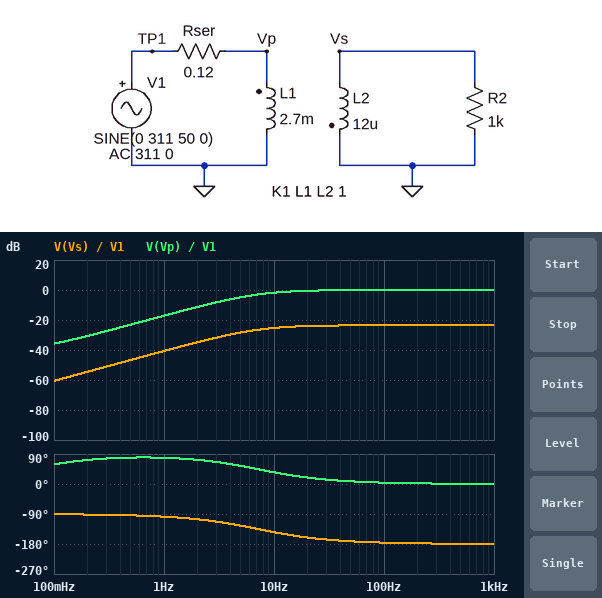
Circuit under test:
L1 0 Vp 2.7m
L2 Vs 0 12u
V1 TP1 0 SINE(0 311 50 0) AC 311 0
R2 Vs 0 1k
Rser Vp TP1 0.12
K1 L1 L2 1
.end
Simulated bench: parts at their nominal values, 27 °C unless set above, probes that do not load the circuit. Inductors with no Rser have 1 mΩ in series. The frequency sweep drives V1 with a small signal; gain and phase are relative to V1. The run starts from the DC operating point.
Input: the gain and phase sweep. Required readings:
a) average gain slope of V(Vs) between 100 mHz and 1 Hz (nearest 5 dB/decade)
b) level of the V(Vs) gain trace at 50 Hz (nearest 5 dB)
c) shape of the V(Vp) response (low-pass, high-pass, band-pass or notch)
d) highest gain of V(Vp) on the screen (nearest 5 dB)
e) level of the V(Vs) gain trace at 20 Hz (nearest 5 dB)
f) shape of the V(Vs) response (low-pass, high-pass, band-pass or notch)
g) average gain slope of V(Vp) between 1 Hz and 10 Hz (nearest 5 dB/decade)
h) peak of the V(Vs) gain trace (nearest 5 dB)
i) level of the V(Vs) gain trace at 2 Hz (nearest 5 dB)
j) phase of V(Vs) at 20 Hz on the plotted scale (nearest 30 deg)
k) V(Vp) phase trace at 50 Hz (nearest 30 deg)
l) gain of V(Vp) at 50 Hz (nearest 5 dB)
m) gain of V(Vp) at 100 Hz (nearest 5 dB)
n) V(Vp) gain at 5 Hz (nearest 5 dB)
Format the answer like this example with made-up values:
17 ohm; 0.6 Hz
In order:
20 dB/decade; -25 dB; high-pass; 0 dB; -25 dB; high-pass; 15 dB/decade; -25 dB; -35 dB; -150 deg; 0 deg; 0 dB; 0 dB; -5 dB
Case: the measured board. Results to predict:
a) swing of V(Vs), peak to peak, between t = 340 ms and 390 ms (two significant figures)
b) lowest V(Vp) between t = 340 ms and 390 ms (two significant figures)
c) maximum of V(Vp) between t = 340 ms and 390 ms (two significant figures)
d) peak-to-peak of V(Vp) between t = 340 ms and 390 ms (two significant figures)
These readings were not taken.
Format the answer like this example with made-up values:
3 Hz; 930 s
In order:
41 V; -310 V; 310 V; 620 V
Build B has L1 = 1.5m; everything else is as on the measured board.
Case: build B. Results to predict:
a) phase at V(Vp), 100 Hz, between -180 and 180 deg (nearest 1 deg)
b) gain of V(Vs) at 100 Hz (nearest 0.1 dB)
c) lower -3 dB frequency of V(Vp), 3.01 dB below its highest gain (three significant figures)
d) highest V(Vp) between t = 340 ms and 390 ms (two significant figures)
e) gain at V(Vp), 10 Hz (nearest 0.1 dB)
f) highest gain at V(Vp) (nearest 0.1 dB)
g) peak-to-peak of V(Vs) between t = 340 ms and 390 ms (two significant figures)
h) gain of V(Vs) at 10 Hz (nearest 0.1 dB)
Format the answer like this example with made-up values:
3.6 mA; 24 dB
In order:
7 deg; -21.0 dB; 12.8 Hz; 300 V; -4.2 dB; 0 dB; 54 V; -25.2 dB
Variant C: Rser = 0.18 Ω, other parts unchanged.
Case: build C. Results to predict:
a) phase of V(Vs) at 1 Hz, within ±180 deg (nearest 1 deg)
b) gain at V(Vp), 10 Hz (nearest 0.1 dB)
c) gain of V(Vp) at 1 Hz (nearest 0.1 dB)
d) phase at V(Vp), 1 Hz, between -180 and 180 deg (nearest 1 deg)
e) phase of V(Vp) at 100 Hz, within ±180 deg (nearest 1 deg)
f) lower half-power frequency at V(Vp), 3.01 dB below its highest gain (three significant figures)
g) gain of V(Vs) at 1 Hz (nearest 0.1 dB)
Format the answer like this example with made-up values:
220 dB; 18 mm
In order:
-95 deg; -3.3 dB; -20.6 dB; 81 deg; 6 deg; 10.7 Hz; -44.1 dB
